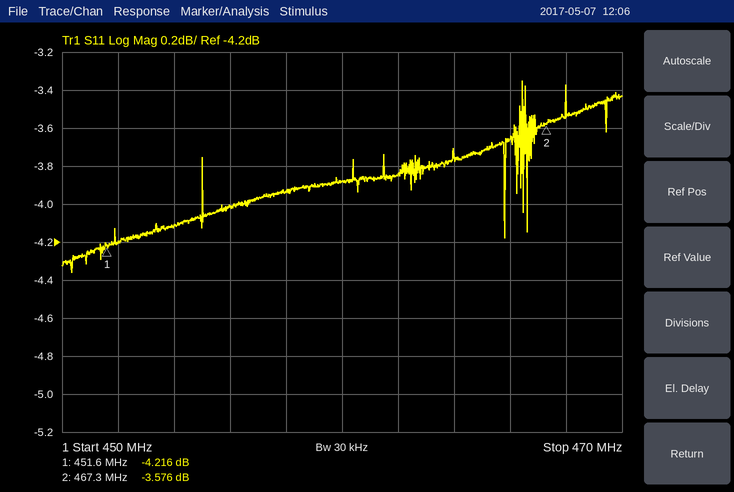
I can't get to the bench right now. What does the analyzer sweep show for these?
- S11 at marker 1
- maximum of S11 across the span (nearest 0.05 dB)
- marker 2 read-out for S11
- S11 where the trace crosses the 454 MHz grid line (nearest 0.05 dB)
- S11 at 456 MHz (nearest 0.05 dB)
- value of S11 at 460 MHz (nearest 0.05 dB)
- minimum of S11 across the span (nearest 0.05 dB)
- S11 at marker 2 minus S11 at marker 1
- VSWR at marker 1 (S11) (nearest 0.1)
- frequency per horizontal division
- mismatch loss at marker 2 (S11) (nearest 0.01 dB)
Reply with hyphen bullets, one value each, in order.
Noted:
- -4.216 dB
- -3.35 dB
- -3.576 dB
- -4.10 dB
- -4.00 dB
- -3.90 dB
- -4.35 dB
- 0.640 dB
- 4.2
- 2 MHz
- 2.51 dB
